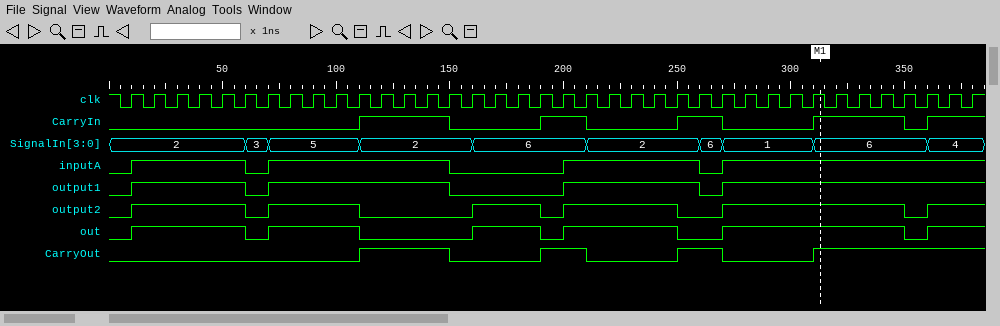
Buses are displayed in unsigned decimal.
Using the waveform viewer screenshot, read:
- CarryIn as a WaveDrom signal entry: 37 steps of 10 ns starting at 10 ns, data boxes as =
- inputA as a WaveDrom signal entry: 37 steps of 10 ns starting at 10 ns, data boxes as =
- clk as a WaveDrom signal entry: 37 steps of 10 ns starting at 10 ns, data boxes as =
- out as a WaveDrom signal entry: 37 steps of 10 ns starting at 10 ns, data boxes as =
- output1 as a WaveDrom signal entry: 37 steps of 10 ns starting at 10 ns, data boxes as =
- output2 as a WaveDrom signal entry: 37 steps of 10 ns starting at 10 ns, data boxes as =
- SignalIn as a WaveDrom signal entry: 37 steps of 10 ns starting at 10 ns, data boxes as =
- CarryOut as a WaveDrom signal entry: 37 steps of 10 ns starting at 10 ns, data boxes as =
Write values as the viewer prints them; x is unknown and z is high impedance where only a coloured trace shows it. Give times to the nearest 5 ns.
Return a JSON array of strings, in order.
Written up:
["{name: 'CarryIn', wave: '0.........1...0...1.0...1.0...1...01.'}", "{name: 'inputA', wave: '1....01.......0....1.....01..........'}", "{name: 'clk', wave: 'p....................................'}", "{name: 'out', wave: '1....01...0....1..01....0.1.......01.'}", "{name: 'output1', wave: '1....01.......0....1.....01..........'}", "{name: 'output2', wave: '1....01...0....1..01....0.1.......01.'}", "{name: 'SignalIn', wave: '=....==...=....=....=....==...=....=.', data: '2 3 5 2 6 2 6 1 6 4'}", "{name: 'CarryOut', wave: '0.........1...0...1.0...1.0...1......'}"]
